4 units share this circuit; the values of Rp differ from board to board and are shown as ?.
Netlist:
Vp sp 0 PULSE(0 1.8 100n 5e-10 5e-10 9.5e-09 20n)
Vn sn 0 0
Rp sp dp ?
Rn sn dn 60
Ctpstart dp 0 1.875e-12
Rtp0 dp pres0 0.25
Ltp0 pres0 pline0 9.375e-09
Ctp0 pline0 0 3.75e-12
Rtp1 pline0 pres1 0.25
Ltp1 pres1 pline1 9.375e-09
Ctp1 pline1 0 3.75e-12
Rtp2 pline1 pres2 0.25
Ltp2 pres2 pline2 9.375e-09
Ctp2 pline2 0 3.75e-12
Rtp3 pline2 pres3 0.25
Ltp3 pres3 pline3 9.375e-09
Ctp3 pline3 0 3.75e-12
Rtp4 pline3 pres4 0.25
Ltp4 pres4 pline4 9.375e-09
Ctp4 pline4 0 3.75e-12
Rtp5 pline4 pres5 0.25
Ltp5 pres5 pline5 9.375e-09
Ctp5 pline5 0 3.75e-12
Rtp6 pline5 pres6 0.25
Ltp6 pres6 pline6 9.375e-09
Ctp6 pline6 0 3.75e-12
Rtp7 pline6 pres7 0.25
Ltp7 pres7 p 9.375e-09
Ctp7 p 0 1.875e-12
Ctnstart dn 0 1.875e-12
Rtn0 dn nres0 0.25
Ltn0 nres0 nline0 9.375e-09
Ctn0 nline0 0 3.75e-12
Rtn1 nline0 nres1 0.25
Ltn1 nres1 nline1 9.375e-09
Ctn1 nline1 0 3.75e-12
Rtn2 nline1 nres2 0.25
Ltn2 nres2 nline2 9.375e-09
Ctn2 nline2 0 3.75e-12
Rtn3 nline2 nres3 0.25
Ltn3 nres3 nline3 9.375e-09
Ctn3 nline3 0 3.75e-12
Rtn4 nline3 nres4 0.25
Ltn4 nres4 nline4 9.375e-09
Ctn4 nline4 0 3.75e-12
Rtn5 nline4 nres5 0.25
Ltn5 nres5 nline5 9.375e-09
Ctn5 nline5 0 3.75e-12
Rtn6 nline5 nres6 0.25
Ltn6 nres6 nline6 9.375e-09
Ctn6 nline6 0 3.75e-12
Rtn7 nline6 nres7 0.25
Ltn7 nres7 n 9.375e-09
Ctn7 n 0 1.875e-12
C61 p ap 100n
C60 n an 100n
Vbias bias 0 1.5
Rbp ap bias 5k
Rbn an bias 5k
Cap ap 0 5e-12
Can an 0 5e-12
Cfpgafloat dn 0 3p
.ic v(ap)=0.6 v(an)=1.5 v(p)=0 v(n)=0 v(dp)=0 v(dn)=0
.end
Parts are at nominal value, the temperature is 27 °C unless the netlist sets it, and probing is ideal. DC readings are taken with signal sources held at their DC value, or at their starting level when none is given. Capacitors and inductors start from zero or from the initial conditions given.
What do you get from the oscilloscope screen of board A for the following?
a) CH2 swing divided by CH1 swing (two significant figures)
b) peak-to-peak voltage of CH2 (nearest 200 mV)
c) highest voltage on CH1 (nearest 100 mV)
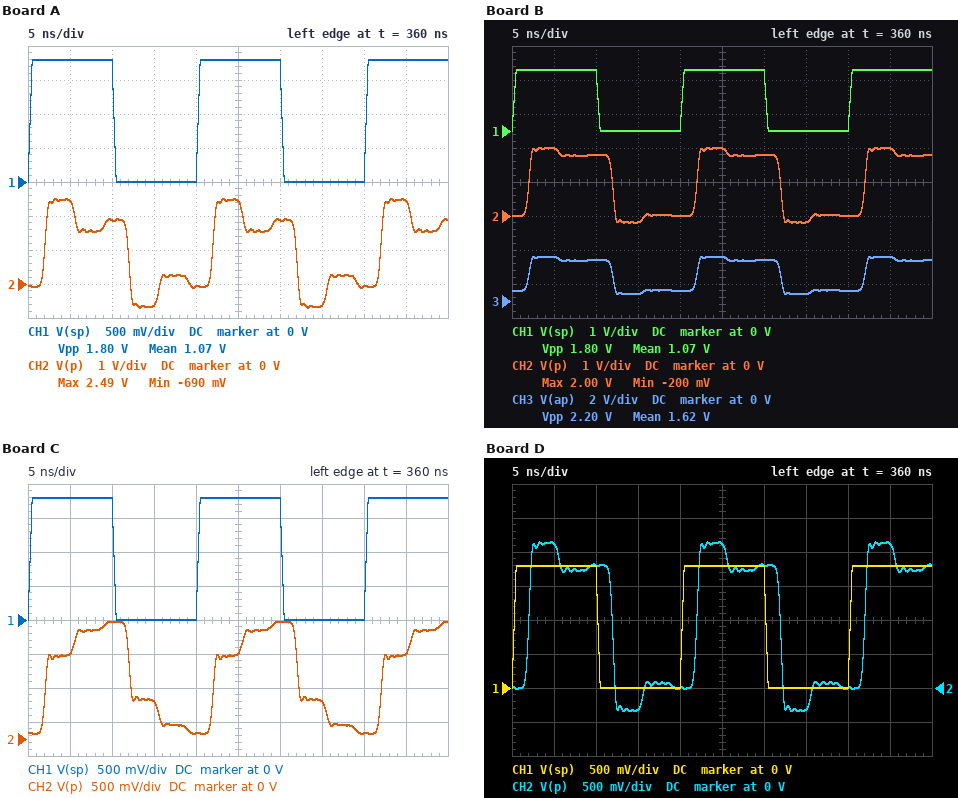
1.8
3.2 V
1.8 V
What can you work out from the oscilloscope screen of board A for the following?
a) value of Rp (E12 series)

22 Ω
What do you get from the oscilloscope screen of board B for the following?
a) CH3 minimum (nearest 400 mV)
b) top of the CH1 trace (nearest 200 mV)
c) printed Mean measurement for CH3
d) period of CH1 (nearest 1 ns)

400 mV
1.8 V
1.62 V
20 ns
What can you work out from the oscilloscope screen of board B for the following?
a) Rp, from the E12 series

39 Ω
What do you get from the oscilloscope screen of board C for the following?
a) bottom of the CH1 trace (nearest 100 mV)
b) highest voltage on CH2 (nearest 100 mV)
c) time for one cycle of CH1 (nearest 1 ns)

0 V
1.7 V
20 ns
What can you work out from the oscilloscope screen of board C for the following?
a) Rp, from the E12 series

100 Ω
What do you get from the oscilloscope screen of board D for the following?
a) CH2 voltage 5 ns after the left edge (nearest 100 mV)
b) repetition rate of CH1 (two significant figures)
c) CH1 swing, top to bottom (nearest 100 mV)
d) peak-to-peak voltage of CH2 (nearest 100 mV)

2.1 V
50 MHz
1.8 V
2.5 V
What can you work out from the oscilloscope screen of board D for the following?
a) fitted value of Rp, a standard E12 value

33 Ω
